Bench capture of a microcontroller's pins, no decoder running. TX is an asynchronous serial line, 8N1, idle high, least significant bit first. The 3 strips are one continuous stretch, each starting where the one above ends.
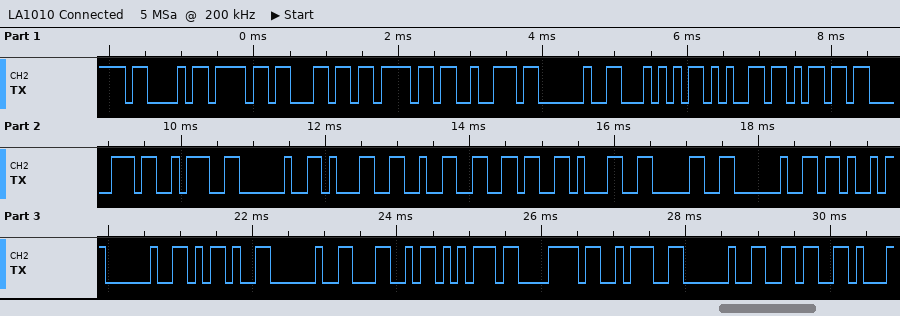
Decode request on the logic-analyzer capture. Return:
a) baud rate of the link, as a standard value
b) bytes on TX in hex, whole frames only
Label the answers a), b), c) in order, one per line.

a) 9600 baud
b) 43 6F 6C 6F 72 20 54 65 6D 70 3A 20 31 32 36 31 30 20 4B 20 2D 20 4C 75 78 3A 20 36
